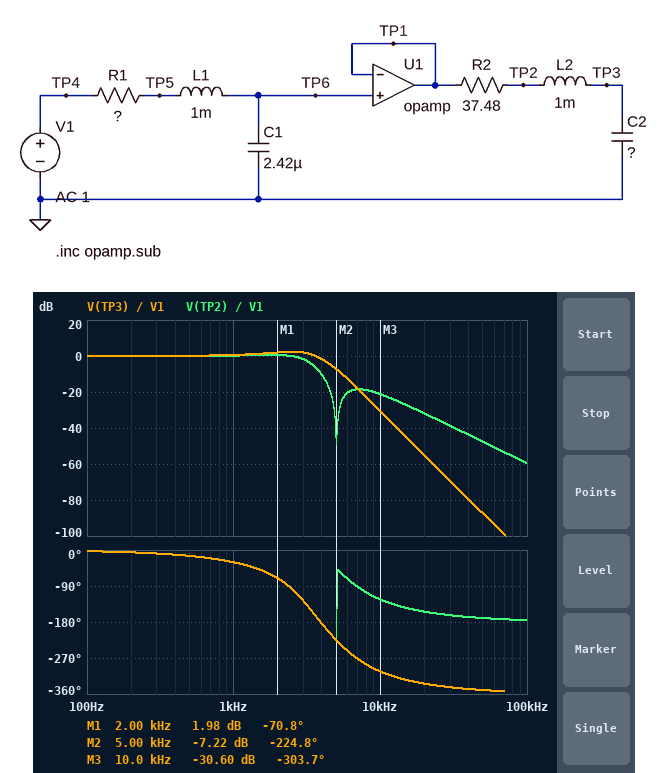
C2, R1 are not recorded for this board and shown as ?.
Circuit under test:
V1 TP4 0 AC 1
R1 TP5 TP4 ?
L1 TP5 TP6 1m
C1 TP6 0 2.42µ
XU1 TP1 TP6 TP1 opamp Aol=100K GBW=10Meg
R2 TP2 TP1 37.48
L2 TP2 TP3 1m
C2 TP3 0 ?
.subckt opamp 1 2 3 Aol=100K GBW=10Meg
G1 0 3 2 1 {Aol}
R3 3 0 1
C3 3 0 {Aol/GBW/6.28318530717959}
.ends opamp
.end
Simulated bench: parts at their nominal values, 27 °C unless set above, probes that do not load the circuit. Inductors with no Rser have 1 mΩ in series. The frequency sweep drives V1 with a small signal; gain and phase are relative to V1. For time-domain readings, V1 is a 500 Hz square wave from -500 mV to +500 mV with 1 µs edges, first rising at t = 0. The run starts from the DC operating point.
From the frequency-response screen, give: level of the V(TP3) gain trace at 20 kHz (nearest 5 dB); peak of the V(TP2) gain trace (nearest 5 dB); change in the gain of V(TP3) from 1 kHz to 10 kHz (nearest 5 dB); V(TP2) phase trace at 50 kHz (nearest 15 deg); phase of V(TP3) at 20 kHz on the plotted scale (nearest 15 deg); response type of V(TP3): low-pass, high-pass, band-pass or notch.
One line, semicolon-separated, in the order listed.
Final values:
-55 dB; 0 dB; -30 dB; -165 deg; -330 deg; low-pass
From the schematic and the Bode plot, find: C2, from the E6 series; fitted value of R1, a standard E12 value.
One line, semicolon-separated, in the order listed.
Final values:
1 µF; 18 Ω
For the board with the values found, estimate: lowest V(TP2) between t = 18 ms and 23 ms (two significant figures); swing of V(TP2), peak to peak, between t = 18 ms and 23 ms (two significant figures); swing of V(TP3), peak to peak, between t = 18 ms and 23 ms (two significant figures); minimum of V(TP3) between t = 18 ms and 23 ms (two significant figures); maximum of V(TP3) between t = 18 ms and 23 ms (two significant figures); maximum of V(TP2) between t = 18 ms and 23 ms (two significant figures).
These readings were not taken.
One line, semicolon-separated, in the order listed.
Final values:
-670 mV; 1.3 V; 1.5 V; -760 mV; 760 mV; 670 mV
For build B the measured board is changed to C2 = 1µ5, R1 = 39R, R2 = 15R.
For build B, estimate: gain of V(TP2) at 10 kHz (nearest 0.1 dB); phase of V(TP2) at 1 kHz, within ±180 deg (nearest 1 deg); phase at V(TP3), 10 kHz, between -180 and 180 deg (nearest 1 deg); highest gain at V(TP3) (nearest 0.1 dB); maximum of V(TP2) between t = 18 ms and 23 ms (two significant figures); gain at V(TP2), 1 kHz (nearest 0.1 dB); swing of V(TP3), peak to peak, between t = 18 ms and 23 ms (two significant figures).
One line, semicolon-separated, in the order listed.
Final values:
-20.7 dB; -42 deg; 51 deg; 0 dB; 520 mV; -0.8 dB; 1.1 V
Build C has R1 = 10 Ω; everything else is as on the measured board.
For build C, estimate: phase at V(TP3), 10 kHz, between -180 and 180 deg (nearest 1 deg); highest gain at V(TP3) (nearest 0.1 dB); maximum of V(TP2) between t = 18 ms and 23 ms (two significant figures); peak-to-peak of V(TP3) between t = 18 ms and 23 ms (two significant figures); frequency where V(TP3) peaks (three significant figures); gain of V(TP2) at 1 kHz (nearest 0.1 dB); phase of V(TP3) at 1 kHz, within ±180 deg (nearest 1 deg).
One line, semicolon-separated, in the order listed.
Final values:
49 deg; 6.8 dB; 800 mV; 2.0 V; 3.02 kHz; 0.5 dB; -23 deg
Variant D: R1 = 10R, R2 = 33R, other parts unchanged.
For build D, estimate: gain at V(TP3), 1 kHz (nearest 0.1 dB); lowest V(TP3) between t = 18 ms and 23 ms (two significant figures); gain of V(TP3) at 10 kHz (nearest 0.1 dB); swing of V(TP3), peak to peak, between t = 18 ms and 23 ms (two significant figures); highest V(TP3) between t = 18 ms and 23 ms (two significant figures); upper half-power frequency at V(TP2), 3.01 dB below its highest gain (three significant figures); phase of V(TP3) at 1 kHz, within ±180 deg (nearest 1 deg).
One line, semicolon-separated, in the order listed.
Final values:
0.9 dB; -1.0 V; -29.9 dB; 2.1 V; 1.0 V; 3.45 kHz; -22 deg
